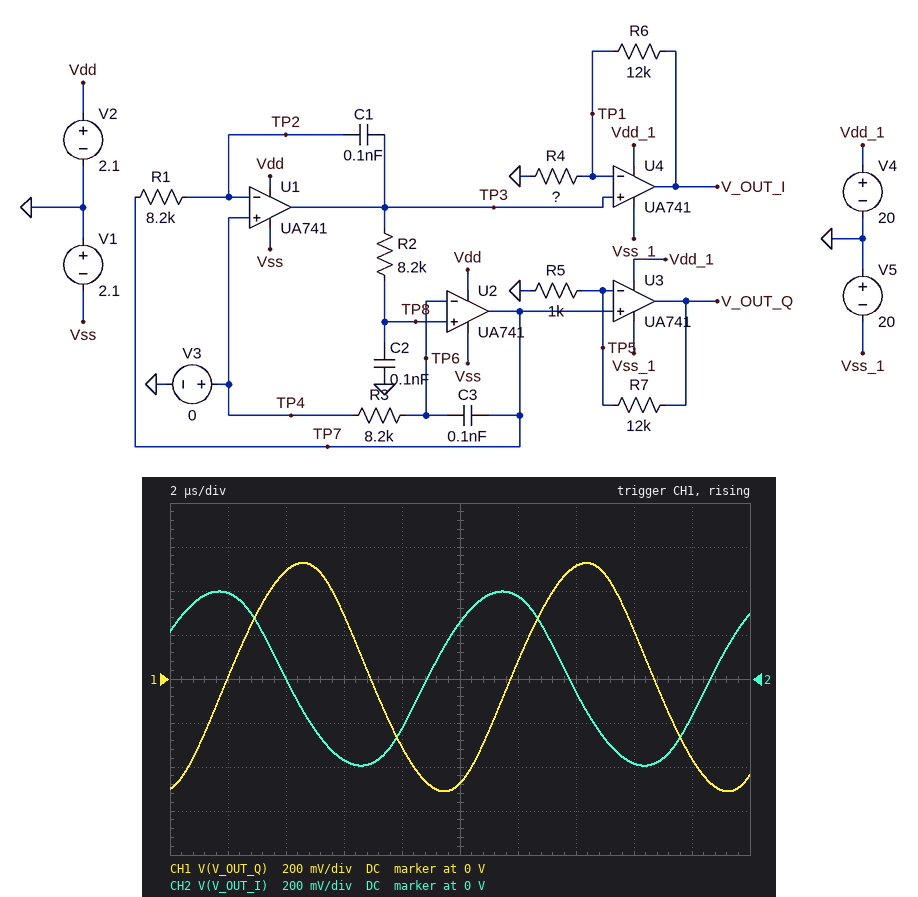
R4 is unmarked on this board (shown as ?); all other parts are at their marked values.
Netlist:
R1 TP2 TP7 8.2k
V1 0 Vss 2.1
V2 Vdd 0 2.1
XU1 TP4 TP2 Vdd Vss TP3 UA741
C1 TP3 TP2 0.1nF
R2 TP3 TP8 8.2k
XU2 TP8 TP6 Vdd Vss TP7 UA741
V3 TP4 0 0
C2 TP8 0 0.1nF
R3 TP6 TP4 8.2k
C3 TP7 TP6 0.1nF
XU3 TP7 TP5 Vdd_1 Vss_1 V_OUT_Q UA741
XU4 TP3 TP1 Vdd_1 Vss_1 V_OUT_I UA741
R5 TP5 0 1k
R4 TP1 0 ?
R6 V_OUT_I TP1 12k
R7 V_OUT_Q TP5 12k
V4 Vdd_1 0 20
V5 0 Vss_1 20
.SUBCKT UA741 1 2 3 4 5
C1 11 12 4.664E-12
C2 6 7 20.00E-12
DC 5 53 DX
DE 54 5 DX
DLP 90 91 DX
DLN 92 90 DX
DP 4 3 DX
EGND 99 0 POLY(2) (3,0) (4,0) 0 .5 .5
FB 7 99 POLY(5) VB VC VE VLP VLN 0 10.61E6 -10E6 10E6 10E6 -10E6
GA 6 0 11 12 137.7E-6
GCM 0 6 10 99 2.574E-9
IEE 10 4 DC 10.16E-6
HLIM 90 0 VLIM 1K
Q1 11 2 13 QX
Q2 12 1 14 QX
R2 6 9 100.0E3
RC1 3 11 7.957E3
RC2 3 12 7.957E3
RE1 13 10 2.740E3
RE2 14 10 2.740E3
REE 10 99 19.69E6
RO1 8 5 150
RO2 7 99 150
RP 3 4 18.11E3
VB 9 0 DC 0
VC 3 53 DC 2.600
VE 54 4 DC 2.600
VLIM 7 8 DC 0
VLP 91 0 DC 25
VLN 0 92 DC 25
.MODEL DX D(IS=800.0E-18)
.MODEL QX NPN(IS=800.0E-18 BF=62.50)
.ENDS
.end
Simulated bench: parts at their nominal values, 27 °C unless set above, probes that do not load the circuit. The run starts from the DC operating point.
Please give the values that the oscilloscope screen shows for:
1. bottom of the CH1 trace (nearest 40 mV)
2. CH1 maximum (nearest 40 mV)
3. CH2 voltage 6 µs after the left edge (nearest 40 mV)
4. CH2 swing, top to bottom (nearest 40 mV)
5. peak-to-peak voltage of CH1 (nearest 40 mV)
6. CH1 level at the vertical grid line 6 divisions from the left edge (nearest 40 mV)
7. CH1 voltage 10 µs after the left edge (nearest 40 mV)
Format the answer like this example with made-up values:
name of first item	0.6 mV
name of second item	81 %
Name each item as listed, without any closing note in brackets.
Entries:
bottom of the CH1 trace	-520 mV
CH1 maximum	520 mV
CH2 voltage 6 µs after the left edge	-360 mV
CH2 swing, top to bottom	800 mV
peak-to-peak voltage of CH1	1.04 V
CH1 level at the vertical grid line 6 divisions from the left edge	80 mV
CH1 voltage 10 µs after the left edge	-480 mV
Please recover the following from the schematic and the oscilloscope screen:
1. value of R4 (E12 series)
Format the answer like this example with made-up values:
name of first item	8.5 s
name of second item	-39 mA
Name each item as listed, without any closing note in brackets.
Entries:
value of R4	1.8 kΩ
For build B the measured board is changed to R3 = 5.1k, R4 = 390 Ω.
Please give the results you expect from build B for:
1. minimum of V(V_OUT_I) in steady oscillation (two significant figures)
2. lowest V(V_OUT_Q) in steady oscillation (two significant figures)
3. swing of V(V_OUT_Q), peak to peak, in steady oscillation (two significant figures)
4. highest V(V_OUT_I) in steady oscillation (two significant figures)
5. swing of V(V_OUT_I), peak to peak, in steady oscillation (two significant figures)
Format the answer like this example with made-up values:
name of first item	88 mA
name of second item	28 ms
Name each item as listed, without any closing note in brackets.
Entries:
minimum of V(V_OUT_I) in steady oscillation	-700 mV
lowest V(V_OUT_Q) in steady oscillation	-630 mV
swing of V(V_OUT_Q), peak to peak, in steady oscillation	1.3 V
highest V(V_OUT_I) in steady oscillation	730 mV
swing of V(V_OUT_I), peak to peak, in steady oscillation	1.4 V
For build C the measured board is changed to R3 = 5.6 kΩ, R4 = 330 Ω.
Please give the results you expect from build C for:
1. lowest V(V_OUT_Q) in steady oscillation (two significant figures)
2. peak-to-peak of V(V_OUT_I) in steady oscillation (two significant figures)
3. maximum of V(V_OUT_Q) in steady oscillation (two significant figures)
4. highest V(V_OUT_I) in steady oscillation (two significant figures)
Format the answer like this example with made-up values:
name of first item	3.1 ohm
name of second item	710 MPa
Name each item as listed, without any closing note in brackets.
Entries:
lowest V(V_OUT_Q) in steady oscillation	-620 mV
peak-to-peak of V(V_OUT_I) in steady oscillation	1.4 V
maximum of V(V_OUT_Q) in steady oscillation	630 mV
highest V(V_OUT_I) in steady oscillation	730 mV
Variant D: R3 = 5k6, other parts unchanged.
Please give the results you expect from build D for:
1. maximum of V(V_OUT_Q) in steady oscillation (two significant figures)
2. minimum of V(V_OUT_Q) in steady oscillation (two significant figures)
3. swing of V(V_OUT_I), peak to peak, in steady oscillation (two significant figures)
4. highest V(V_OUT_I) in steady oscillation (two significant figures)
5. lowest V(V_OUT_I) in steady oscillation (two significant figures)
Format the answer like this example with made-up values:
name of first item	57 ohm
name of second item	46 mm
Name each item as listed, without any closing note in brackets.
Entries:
maximum of V(V_OUT_Q) in steady oscillation	630 mV
minimum of V(V_OUT_Q) in steady oscillation	-620 mV
swing of V(V_OUT_I), peak to peak, in steady oscillation	910 mV
highest V(V_OUT_I) in steady oscillation	460 mV
lowest V(V_OUT_I) in steady oscillation	-450 mV
